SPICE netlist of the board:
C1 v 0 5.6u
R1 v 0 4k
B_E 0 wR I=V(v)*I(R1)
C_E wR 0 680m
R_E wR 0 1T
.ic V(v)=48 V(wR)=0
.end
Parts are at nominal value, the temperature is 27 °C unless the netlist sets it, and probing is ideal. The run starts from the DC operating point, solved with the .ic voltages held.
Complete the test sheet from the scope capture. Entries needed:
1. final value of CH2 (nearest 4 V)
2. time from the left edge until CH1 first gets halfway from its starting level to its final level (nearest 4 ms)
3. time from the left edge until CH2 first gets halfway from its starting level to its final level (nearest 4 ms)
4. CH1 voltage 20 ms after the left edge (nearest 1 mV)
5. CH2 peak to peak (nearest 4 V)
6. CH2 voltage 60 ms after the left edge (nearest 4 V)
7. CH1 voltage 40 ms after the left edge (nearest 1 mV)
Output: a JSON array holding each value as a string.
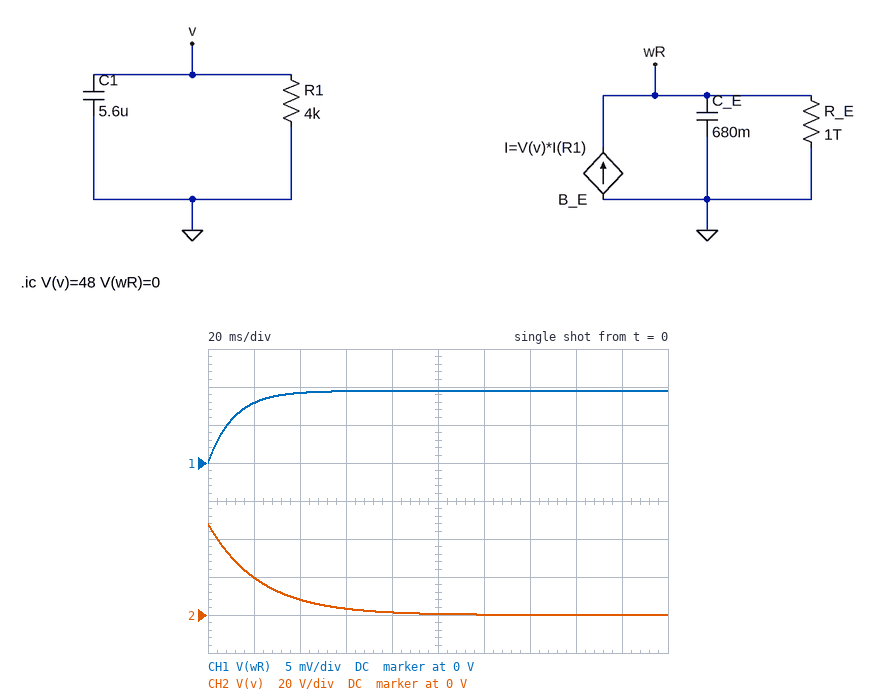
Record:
["0 V", "8 ms", "16 ms", "8 mV", "48 V", "4 V", "9 mV"]
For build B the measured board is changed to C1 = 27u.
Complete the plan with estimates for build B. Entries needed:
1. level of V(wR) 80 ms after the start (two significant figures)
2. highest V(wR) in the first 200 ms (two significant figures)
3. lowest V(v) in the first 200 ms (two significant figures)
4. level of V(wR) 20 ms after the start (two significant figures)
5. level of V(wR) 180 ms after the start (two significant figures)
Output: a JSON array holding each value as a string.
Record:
["35 mV", "45 mV", "7.5 V", "14 mV", "44 mV"]
